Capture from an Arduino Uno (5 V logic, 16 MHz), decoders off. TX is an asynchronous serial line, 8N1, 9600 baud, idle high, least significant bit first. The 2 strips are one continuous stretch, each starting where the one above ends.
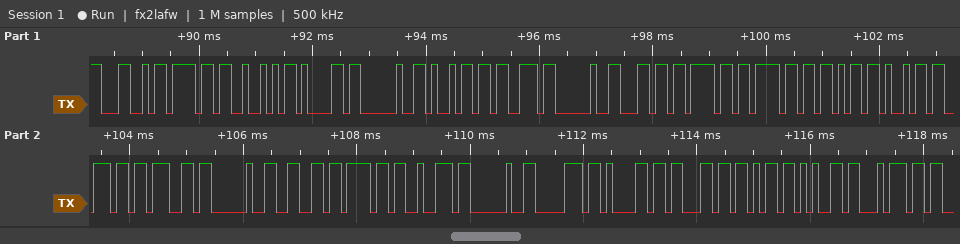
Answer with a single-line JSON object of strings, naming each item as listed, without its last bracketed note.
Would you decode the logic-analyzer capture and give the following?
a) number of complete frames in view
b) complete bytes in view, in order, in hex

{"number of complete frames in view": "26", "complete bytes in view, in order, in hex": "4C 6F 52 61 20 69 73 20 6C 6F 6F 6B 69 6E 67 20 66 6F 72 20 70 61 63 6B 65 74"}
